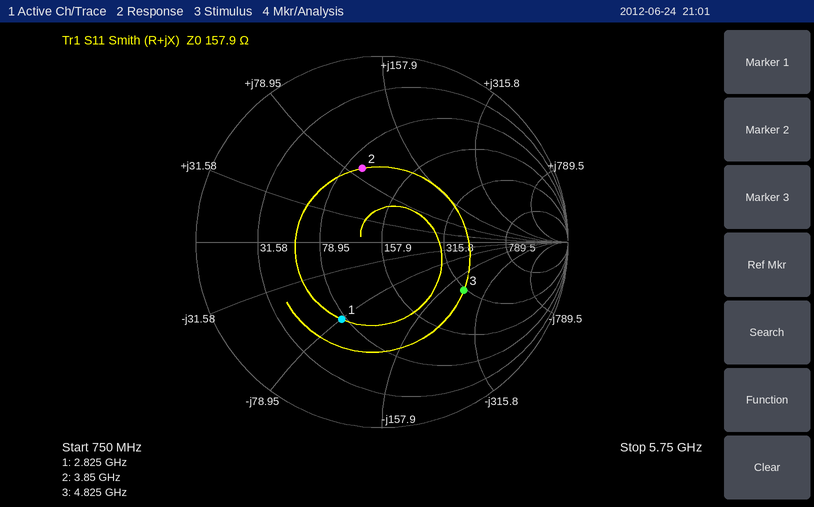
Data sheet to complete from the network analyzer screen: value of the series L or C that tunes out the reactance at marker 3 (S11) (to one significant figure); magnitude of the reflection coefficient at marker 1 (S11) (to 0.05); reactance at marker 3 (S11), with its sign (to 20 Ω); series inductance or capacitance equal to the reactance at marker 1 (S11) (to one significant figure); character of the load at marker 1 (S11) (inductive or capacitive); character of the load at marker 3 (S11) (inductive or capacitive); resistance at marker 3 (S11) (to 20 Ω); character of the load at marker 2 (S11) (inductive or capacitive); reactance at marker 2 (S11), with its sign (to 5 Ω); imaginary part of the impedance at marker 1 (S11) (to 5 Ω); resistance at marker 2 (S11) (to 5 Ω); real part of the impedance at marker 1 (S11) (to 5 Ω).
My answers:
7 nH
0.45
-220 Ω
700 fF
capacitive
capacitive
300 Ω
inductive
+90 Ω
-80 Ω
95 Ω
75 Ω
